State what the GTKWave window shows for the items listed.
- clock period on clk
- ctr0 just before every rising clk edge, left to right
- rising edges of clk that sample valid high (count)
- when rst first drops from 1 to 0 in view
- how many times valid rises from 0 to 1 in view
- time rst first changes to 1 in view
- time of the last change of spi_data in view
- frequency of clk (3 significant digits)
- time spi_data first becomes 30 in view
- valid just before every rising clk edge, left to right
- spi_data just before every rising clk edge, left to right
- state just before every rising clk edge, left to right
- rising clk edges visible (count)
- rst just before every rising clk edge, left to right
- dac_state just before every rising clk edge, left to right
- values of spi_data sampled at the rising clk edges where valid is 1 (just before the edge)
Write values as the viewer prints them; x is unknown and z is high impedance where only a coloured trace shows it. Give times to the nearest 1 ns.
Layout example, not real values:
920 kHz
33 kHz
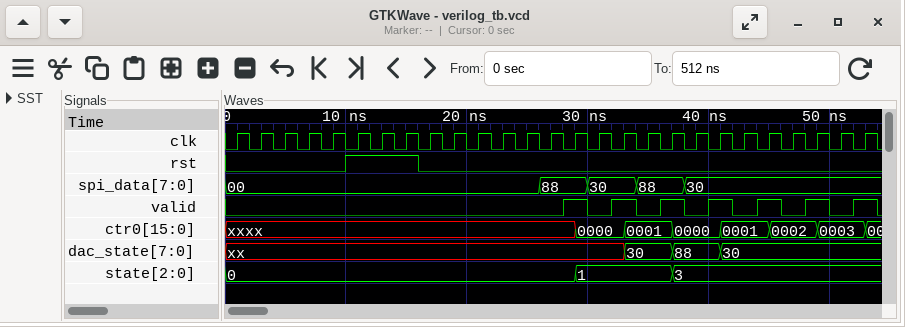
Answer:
2 ns
xxxx, xxxx, xxxx, xxxx, xxxx, xxxx, xxxx, xxxx, xxxx, xxxx, xxxx, xxxx, xxxx, xxxx, xxxx, 0000, 0000, 0001, 0001, 0000, 0000, 0001, 0001, 0002, 0002, 0003, 0003
7
16 ns
7
10 ns
38 ns
500 MHz
30 ns
0 0 0 0 0 0 0 0 0 0 0 0 0 0 1 0 1 0 1 0 1 0 1 0 1 0 1
00, 00, 00, 00, 00, 00, 00, 00, 00, 00, 00, 00, 00, 88, 88, 30, 30, 88, 88, 30, 30, 30, 30, 30, 30, 30, 30
0, 0, 0, 0, 0, 0, 0, 0, 0, 0, 0, 0, 0, 0, 0, 1, 1, 1, 1, 3, 3, 3, 3, 3, 3, 3, 3
27
0 0 0 0 0 1 1 1 0 0 0 0 0 0 0 0 0 0 0 0 0 0 0 0 0 0 0
xx, xx, xx, xx, xx, xx, xx, xx, xx, xx, xx, xx, xx, xx, xx, xx, xx, 30, 30, 88, 88, 30, 30, 30, 30, 30, 30
88, 30, 88, 30, 30, 30, 30
